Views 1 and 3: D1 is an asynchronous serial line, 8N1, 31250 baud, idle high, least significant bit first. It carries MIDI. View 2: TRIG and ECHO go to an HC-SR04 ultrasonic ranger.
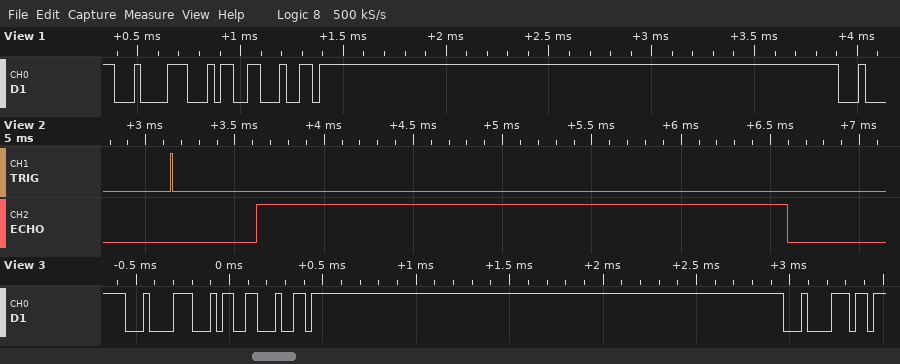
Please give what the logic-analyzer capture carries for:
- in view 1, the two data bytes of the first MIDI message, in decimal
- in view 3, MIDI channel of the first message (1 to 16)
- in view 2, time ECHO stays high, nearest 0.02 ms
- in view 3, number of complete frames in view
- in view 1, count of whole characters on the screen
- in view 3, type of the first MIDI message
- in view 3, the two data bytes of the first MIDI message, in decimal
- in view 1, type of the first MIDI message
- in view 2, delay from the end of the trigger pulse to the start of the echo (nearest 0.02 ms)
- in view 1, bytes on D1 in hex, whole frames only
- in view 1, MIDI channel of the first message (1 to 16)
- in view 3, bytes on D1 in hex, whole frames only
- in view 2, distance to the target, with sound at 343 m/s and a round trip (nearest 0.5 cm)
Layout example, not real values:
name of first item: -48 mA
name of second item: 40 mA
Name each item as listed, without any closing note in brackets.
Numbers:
in view 1, the two data bytes of the first MIDI message, in decimal: 52, 100
in view 3, MIDI channel of the first message: 5
in view 2, time ECHO stays high, nearest 0.02 ms: 2.98 ms
in view 3, number of complete frames in view: 4
in view 1, count of whole characters on the screen: 3
in view 3, type of the first MIDI message: Note Off
in view 3, the two data bytes of the first MIDI message, in decimal: 52, 100
in view 1, type of the first MIDI message: Note Off
in view 2, delay from the end of the trigger pulse to the start of the echo: 0.46 ms
in view 1, bytes on D1 in hex, whole frames only: 0x84 0x34 0x64
in view 1, MIDI channel of the first message: 5
in view 3, bytes on D1 in hex, whole frames only: 84 34 64 84
in view 2, distance to the target, with sound at 343 m/s and a round trip: 51 cm
